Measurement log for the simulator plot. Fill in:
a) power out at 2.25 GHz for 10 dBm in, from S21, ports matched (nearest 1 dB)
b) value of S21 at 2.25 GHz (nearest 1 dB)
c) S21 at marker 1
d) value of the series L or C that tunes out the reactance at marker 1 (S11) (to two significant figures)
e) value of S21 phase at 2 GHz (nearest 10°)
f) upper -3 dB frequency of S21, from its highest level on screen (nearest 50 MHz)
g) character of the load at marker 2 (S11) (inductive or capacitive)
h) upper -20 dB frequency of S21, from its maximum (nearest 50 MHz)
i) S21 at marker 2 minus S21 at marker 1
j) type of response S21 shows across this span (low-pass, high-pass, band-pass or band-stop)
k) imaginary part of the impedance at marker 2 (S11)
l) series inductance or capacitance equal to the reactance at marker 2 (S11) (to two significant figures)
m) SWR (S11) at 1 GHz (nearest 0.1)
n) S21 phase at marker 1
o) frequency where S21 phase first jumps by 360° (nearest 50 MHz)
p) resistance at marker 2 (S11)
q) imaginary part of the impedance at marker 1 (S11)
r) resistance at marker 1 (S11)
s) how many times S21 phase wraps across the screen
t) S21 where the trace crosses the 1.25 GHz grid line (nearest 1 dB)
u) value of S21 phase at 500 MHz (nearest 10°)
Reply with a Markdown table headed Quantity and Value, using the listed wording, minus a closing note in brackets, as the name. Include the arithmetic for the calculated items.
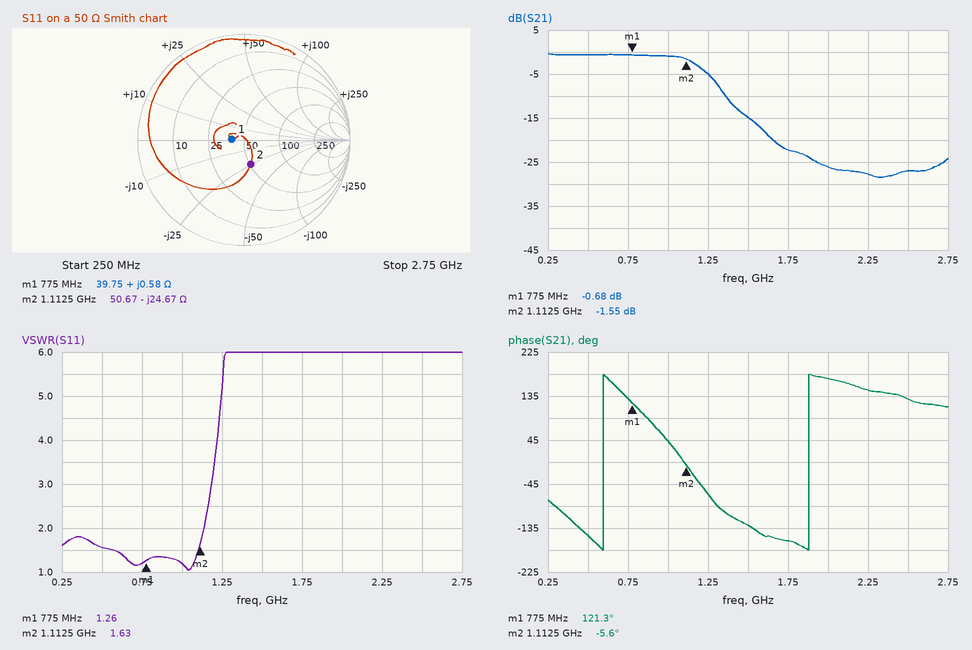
| Quantity | Value |
|---|---|
| power out at 2.25 GHz for 10 dBm in, from S21, ports matched | 10 dBm + (-28 dB) = -18 dBm |
| value of S21 at 2.25 GHz | -28 dB |
| S21 at marker 1 | -0.68 dB |
| value of the series L or C that tunes out the reactance at marker 1 (S11) | C = 1/(2π × 775 MHz × 0.58 Ω) ≈ 354 pF, so 350 pF to two significant figures |
| value of S21 phase at 2 GHz | 170° |
| upper -3 dB frequency of S21, from its highest level on screen | 1.20 GHz |
| character of the load at marker 2 (S11) | capacitive |
| upper -20 dB frequency of S21, from its maximum | 1.65 GHz |
| S21 at marker 2 minus S21 at marker 1 | -1.55 − (-0.68) = -0.87 dB |
| type of response S21 shows across this span | low-pass |
| imaginary part of the impedance at marker 2 | -24.67 Ω |
| series inductance or capacitance equal to the reactance at marker 2 (S11) | C = 1/(2π × 1.1125 GHz × 24.67 Ω) ≈ 5.8 pF |
| SWR (S11) at 1 GHz | 1.2 |
| S21 phase at marker 1 | 121.3° |
| frequency where S21 phase first jumps by 360° | 600 MHz |
| resistance at marker 2 | 50.67 Ω |
| imaginary part of the impedance at marker 1 | +0.58 Ω |
| resistance at marker 1 | 39.75 Ω |
| how many times S21 phase wraps across the screen | 2 |
| S21 where the trace crosses the 1.25 GHz grid line | -5 dB |
| value of S21 phase at 500 MHz | -150° |
